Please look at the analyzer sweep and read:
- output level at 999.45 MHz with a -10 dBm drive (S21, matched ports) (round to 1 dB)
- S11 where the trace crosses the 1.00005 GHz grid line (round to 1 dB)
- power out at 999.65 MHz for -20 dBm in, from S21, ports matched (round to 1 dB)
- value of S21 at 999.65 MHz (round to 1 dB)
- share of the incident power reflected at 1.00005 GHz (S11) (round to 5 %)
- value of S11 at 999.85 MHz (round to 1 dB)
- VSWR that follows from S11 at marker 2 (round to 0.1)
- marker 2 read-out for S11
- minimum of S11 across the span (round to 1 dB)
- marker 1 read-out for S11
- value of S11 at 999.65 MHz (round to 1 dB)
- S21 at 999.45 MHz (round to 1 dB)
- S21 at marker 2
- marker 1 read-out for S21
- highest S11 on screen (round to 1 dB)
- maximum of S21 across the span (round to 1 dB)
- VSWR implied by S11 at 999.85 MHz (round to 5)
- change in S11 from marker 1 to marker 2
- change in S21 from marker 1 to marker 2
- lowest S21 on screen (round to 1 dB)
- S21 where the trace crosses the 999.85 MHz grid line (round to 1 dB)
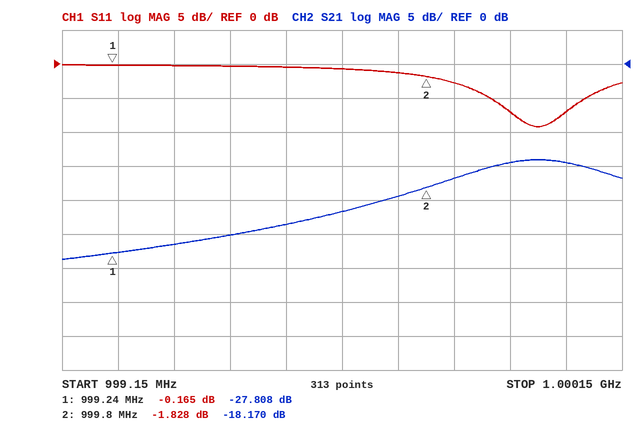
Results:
-35 dBm
-7 dB
-42 dBm
-22 dB
20 %
-3 dB
9.5
-1.828 dB
-9 dB
-0.165 dB
-1 dB
-25 dB
-18.170 dB
-27.808 dB
0 dB
-14 dB
5
-1.663 dB
9.638 dB
-29 dB
-17 dB
